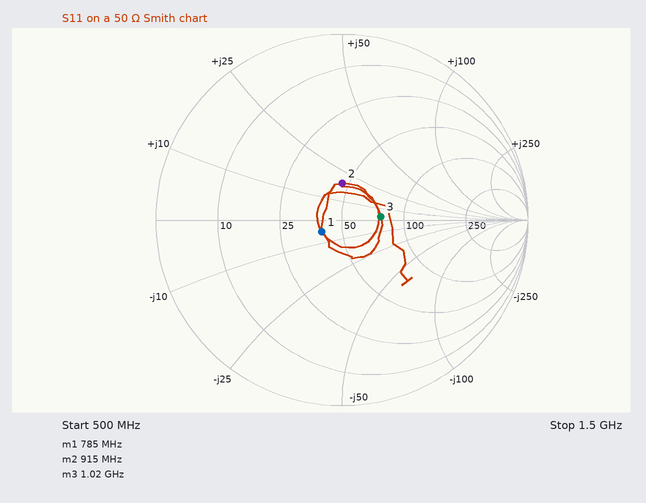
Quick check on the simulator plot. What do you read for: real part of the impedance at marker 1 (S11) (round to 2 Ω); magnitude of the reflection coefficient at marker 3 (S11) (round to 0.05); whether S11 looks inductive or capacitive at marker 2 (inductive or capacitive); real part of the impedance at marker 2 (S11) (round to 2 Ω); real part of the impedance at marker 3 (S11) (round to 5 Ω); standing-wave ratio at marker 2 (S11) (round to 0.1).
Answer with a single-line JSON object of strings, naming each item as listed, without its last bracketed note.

{"real part of the impedance at marker 1 (S11)": "40 Ω", "magnitude of the reflection coefficient at marker 3 (S11)": "0.20", "whether S11 looks inductive or capacitive at marker 2": "inductive", "real part of the impedance at marker 2 (S11)": "46 Ω", "real part of the impedance at marker 3 (S11)": "75 Ω", "standing-wave ratio at marker 2 (S11)": "1.5"}
